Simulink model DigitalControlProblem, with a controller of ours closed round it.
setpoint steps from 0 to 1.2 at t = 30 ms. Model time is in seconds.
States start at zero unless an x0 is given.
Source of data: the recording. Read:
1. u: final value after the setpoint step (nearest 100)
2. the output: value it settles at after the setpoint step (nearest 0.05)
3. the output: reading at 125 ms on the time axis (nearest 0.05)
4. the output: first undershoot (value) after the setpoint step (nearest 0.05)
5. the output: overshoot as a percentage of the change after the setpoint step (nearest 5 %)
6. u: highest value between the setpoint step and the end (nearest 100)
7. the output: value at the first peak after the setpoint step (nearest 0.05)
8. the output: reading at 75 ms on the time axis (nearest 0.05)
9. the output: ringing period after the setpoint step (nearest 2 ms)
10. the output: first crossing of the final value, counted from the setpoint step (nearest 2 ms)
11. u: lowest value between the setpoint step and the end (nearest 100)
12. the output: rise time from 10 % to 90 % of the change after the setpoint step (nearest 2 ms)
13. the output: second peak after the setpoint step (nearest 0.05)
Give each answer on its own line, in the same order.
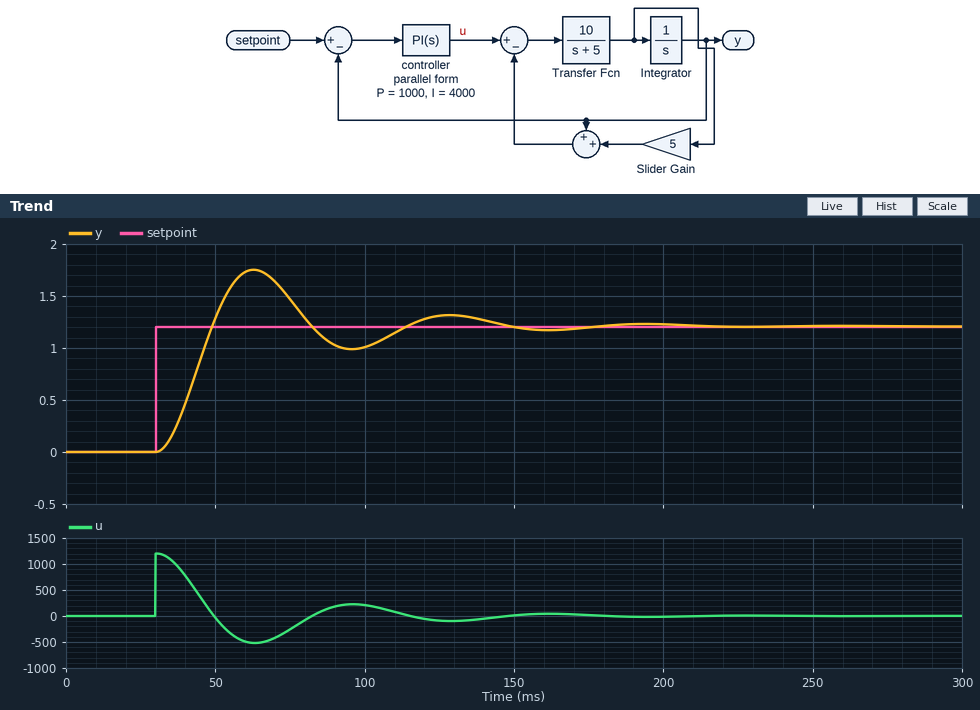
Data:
0
1.20
1.30
1.00
45 %
1200
1.75
1.45
66 ms
18 ms
-500
12 ms
1.30
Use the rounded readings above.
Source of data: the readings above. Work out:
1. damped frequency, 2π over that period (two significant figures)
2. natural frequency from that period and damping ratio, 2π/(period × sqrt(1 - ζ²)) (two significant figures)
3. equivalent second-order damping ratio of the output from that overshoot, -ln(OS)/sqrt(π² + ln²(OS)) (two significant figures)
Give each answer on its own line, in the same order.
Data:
0.095 rad/ms
0.098 rad/ms
0.25
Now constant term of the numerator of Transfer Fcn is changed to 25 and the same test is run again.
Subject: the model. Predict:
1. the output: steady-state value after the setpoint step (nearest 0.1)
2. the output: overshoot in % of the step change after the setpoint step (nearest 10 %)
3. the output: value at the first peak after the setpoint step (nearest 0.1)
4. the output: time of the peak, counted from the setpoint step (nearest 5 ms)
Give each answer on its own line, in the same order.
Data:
1.2
30 %
1.5
20 ms
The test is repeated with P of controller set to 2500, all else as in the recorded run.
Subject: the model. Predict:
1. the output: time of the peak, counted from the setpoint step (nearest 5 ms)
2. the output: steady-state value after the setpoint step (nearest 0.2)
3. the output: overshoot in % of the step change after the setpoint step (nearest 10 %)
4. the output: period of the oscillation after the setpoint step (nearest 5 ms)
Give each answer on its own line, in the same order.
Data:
20 ms
1.2
60 %
40 ms
